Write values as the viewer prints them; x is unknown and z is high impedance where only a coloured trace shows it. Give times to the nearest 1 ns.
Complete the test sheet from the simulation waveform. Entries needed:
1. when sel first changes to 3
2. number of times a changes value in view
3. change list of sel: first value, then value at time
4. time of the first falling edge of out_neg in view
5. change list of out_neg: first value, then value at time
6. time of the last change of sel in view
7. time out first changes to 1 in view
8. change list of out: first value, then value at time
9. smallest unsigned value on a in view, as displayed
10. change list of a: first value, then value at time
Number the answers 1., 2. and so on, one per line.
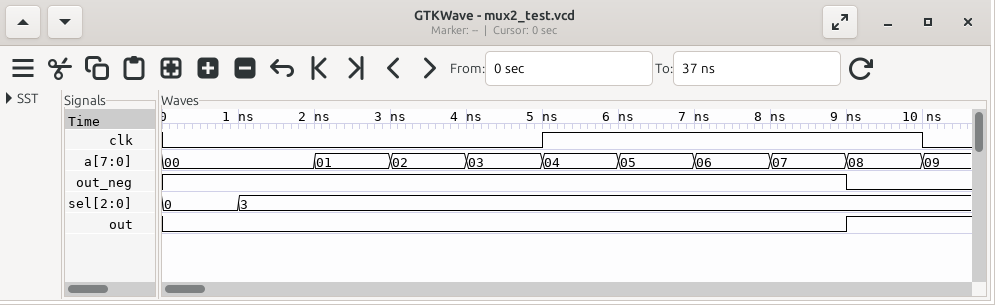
1. 1 ns
2. 9
3. 0, 3 at 1 ns
4. 9 ns
5. 1, 0 at 9 ns
6. 1 ns
7. 9 ns
8. 0, 1 at 9 ns
9. 00
10. 00, 01 at 2 ns, 02 at 3 ns, 03 at 4 ns, 04 at 5 ns, 05 at 6 ns, 06 at 7 ns, 07 at 8 ns, 08 at 9 ns, 09 at 10 ns
